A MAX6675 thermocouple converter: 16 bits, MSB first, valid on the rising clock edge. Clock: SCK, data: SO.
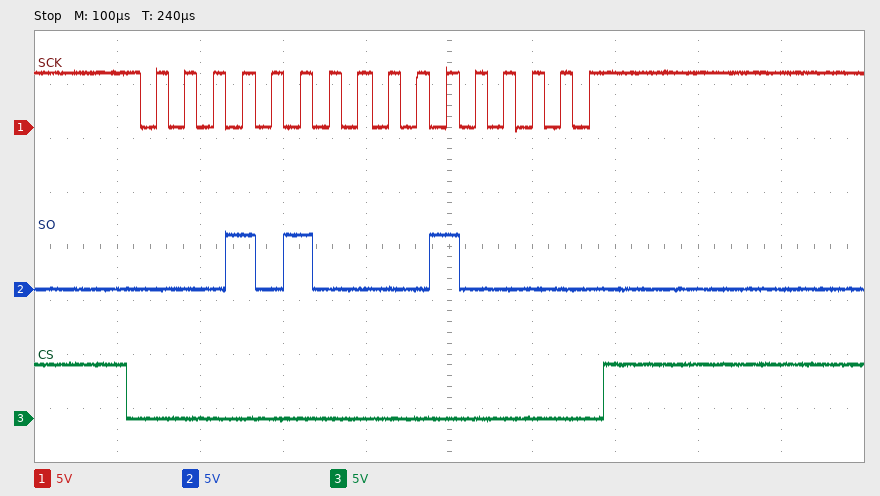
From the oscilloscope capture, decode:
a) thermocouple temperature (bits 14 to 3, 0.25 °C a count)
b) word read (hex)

161.00 °C
0x1420
